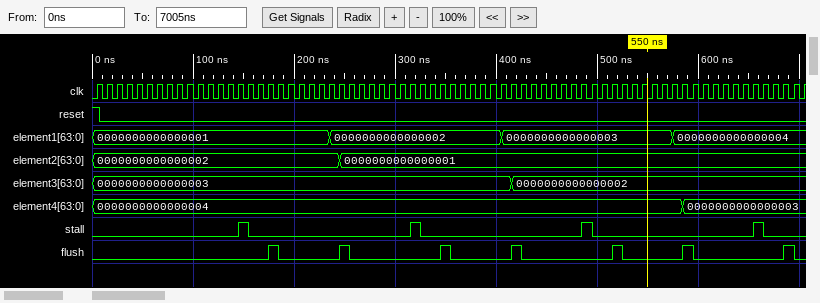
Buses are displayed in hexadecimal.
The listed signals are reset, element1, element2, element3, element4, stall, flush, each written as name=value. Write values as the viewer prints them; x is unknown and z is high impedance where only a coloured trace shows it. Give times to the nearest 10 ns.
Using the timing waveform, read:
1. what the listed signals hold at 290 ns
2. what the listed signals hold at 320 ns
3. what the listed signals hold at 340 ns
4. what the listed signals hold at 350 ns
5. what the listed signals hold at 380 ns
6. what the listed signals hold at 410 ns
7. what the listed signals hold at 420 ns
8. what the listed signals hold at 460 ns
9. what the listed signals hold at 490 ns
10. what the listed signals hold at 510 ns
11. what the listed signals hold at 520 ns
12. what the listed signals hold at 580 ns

reset=0, element1=0000000000000002, element2=0000000000000001, element3=0000000000000003, element4=0000000000000004, stall=0, flush=0
reset=0, element1=0000000000000002, element2=0000000000000001, element3=0000000000000003, element4=0000000000000004, stall=1, flush=0
reset=0, element1=0000000000000002, element2=0000000000000001, element3=0000000000000003, element4=0000000000000004, stall=0, flush=0
reset=0, element1=0000000000000002, element2=0000000000000001, element3=0000000000000003, element4=0000000000000004, stall=0, flush=1
reset=0, element1=0000000000000002, element2=0000000000000001, element3=0000000000000003, element4=0000000000000004, stall=0, flush=0
reset=0, element1=0000000000000003, element2=0000000000000001, element3=0000000000000003, element4=0000000000000004, stall=0, flush=0
reset=0, element1=0000000000000003, element2=0000000000000001, element3=0000000000000002, element4=0000000000000004, stall=0, flush=1
reset=0, element1=0000000000000003, element2=0000000000000001, element3=0000000000000002, element4=0000000000000004, stall=0, flush=0
reset=0, element1=0000000000000003, element2=0000000000000001, element3=0000000000000002, element4=0000000000000004, stall=1, flush=0
reset=0, element1=0000000000000003, element2=0000000000000001, element3=0000000000000002, element4=0000000000000004, stall=0, flush=0
reset=0, element1=0000000000000003, element2=0000000000000001, element3=0000000000000002, element4=0000000000000004, stall=0, flush=1
reset=0, element1=0000000000000004, element2=0000000000000001, element3=0000000000000002, element4=0000000000000004, stall=0, flush=0
